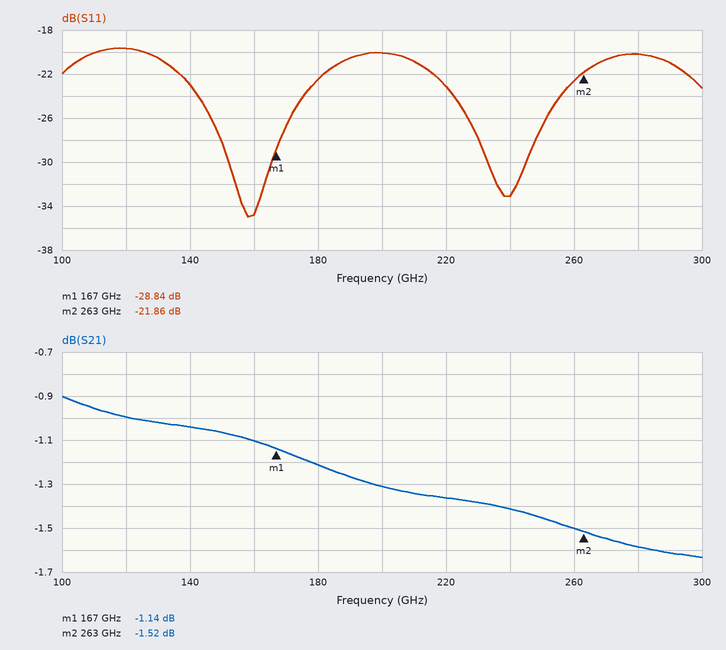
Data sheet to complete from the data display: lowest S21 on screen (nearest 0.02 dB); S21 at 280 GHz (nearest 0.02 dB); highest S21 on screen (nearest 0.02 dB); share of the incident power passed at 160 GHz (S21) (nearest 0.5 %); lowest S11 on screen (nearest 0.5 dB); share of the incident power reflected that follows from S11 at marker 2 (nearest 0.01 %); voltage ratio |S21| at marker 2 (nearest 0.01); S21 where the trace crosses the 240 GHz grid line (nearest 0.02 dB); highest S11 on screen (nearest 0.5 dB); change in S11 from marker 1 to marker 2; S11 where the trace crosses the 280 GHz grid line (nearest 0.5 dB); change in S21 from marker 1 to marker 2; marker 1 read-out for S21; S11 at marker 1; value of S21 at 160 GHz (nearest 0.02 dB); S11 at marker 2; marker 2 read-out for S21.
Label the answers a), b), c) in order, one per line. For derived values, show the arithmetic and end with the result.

a) -1.64 dB
b) -1.58 dB
c) -0.90 dB
d) 10^(-1.1/10) ≈ 77.6 %, so 77.5 % to the nearest 0.5 %
e) -35.0 dB
f) 10^(-21.86/10) ≈ 0.65 %
g) 10^(-1.52/20) ≈ 0.84
h) -1.42 dB
i) -19.5 dB
j) -21.86 − (-28.84) = 6.98 dB
k) -20.0 dB
l) -1.52 − (-1.14) = -0.38 dB
m) -1.14 dB
n) -28.84 dB
o) -1.10 dB
p) -21.86 dB
q) -1.52 dB
